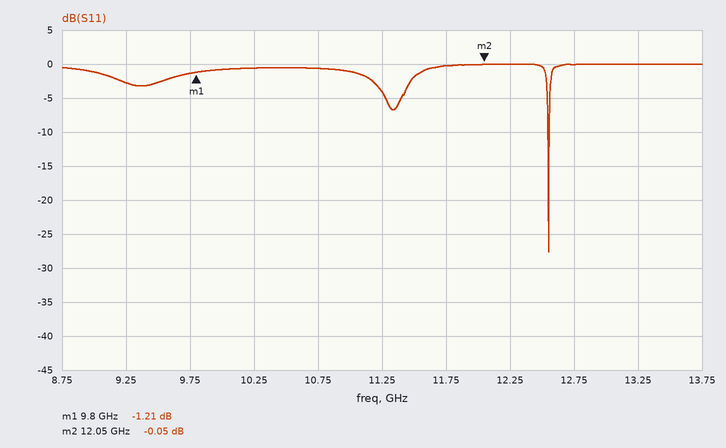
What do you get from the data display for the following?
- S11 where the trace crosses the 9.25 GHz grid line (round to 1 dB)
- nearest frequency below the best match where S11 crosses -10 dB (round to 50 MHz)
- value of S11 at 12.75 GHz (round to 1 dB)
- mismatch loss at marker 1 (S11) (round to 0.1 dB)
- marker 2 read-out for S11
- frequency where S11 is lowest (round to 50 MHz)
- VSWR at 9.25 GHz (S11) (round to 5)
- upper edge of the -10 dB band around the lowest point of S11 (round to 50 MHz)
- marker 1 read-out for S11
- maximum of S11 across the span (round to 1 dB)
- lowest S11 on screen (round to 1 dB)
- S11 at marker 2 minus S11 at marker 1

-3 dB
12.55 GHz
0 dB
6.1 dB
-0.05 dB
12.55 GHz
5
12.55 GHz
-1.21 dB
0 dB
-28 dB
1.16 dB
